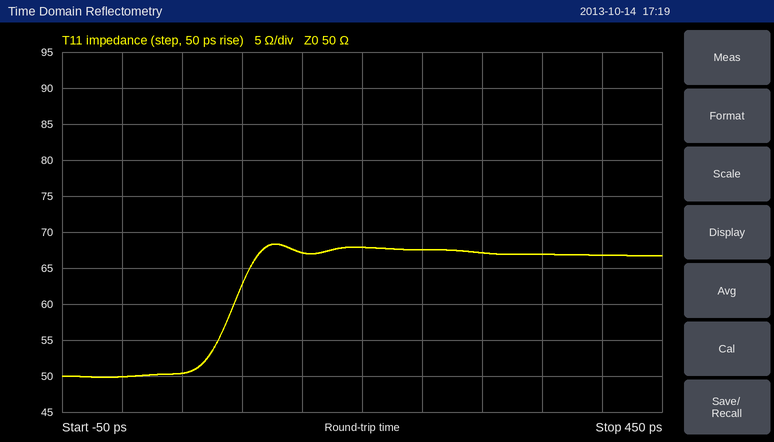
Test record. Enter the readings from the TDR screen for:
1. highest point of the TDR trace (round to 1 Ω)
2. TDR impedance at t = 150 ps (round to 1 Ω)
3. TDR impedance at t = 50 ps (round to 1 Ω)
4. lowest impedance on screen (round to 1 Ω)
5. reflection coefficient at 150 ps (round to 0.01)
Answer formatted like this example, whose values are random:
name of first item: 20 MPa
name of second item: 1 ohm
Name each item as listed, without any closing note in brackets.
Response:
highest point of the TDR trace: 68 Ω
TDR impedance at t = 150 ps: 67 Ω
TDR impedance at t = 50 ps: 50 Ω
lowest impedance on screen: 50 Ω
reflection coefficient at 150 ps: +0.15
